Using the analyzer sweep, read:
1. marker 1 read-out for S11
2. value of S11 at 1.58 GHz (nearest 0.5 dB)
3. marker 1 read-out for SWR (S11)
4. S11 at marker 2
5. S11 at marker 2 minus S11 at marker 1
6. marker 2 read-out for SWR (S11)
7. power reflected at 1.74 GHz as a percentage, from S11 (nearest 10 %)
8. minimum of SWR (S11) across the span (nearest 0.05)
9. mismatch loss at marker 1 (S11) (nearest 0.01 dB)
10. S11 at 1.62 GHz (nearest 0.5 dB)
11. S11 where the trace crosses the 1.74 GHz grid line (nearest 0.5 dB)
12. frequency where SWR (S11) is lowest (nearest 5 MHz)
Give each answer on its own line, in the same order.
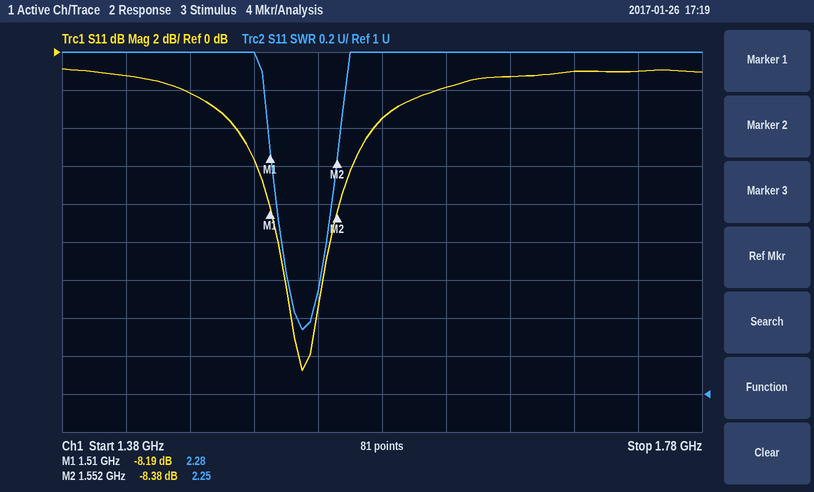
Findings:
-8.19 dB
-3.5 dB
2.28
-8.38 dB
-0.19 dB
2.25
80 %
1.35
0.71 dB
-2.0 dB
-1.0 dB
1.530 GHz
